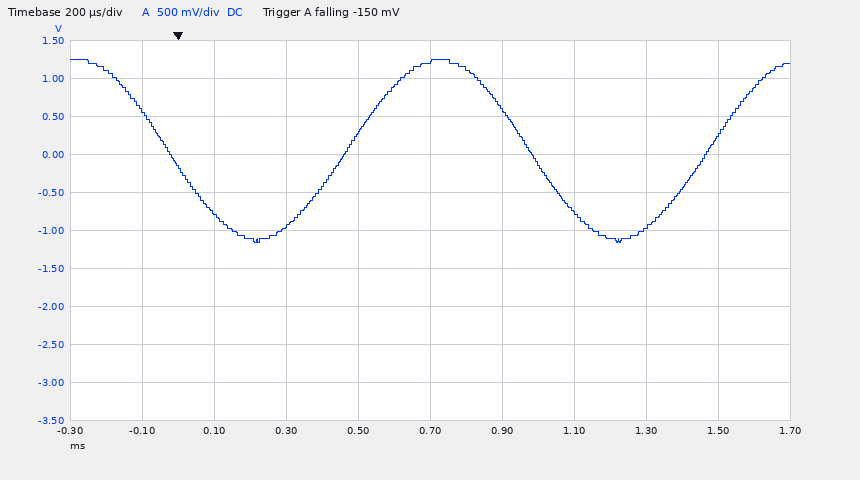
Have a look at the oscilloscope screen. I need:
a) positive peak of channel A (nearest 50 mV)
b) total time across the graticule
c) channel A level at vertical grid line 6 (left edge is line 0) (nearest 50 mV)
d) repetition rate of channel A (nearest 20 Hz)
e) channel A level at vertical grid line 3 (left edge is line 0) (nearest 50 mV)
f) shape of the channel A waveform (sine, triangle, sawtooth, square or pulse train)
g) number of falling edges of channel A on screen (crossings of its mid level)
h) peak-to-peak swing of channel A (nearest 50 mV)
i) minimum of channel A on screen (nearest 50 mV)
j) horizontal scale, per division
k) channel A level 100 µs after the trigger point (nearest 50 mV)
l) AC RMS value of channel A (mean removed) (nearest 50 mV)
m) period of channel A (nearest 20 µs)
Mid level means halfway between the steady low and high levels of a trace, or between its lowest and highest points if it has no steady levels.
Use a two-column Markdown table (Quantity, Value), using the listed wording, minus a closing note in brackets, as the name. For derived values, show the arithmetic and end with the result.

| Quantity | Value |
|---|---|
| positive peak of channel A | 1.25 V |
| total time across the graticule | 2 ms |
| channel A level at vertical grid line 6 (left edge is line 0) | 600 mV |
| repetition rate of channel A | 1 / 1.00 ms ≈ 1.00 kHz |
| channel A level at vertical grid line 3 (left edge is line 0) | -950 mV |
| shape of the channel A waveform | sine |
| number of falling edges of channel A on screen | 2 |
| peak-to-peak swing of channel A | 1.25 V − (-1.15 V) = 2.40 V |
| minimum of channel A on screen | -1.15 V |
| horizontal scale, per division | 200 µs |
| channel A level 100 µs after the trigger point | -800 mV |
| AC RMS value of channel A (mean removed) | 2.40 V / (2√2) ≈ 849 mV, so 850 mV to the nearest 50 mV |
| period of channel A | 1.00 ms |
